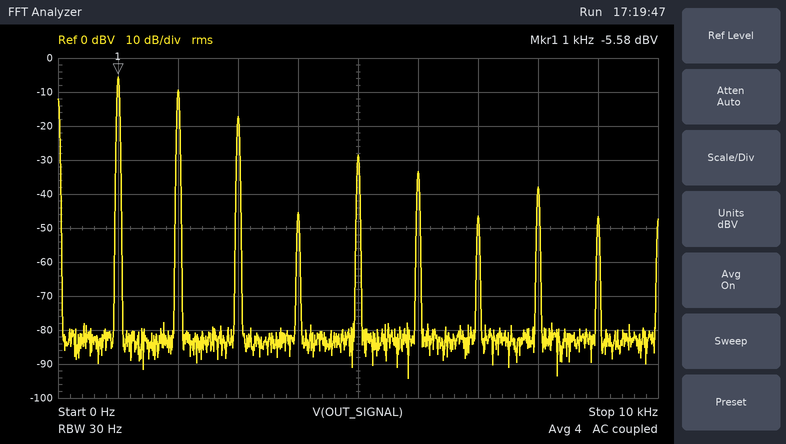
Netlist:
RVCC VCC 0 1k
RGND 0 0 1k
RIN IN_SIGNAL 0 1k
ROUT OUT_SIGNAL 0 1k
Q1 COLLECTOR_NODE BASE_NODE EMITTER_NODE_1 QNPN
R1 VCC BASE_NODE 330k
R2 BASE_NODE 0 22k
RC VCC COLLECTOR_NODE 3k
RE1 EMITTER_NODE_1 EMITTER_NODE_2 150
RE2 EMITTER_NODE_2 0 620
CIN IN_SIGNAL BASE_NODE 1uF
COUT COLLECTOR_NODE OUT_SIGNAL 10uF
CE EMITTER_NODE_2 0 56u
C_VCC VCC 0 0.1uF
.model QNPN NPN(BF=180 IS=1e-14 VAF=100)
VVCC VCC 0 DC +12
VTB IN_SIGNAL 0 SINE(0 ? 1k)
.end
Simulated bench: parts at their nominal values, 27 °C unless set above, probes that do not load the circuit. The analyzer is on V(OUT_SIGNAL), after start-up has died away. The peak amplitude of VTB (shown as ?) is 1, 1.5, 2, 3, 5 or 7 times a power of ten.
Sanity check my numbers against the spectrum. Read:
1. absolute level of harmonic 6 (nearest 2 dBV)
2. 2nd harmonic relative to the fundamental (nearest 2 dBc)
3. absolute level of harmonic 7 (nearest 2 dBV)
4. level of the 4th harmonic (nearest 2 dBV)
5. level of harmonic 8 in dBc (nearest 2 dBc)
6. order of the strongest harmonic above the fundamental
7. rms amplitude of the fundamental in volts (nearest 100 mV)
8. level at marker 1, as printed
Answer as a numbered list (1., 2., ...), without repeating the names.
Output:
1. -34 dBV
2. -4 dBc
3. -46 dBV
4. -46 dBV
5. -32 dBc
6. 2
7. 500 mV
8. -5.58 dBV
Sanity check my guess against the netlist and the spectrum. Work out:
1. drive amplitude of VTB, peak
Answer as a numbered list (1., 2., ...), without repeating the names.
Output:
1. 700 mV
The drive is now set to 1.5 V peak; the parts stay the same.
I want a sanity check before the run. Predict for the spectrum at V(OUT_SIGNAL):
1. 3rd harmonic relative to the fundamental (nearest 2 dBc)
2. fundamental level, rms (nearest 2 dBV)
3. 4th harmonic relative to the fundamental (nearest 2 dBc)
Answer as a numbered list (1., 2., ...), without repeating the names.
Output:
1. -10 dBc
2. 0 dBV
3. -26 dBc
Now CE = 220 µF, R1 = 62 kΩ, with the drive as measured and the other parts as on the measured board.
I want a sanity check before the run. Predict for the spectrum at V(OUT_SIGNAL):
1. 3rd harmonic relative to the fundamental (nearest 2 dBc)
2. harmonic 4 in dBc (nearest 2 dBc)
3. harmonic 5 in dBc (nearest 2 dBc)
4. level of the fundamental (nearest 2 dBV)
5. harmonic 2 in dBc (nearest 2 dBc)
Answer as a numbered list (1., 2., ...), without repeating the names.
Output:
1. -20 dBc
2. -34 dBc
3. -40 dBc
4. 4 dBV
5. -14 dBc
